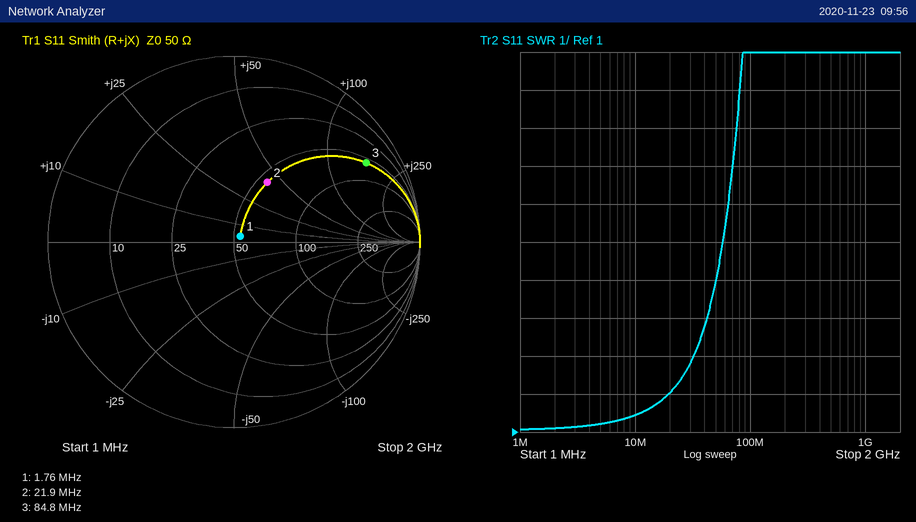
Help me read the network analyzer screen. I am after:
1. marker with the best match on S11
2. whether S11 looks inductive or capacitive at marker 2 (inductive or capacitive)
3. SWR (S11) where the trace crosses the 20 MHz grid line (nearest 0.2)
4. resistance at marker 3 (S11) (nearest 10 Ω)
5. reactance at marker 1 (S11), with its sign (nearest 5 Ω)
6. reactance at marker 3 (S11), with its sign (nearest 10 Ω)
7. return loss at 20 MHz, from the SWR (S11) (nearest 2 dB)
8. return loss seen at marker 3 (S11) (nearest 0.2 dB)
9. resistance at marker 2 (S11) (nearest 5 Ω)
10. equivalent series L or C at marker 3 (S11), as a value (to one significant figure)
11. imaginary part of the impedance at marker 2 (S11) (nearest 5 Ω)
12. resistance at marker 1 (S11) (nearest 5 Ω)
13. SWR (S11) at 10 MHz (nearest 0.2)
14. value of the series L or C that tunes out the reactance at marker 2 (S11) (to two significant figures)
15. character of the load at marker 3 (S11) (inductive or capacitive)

marker 1
inductive
2.0
60 Ω
+5 Ω
+160 Ω
10 dB
1.6 dB
55 Ω
300 nH
+40 Ω
55 Ω
1.4
180 pF
inductive
